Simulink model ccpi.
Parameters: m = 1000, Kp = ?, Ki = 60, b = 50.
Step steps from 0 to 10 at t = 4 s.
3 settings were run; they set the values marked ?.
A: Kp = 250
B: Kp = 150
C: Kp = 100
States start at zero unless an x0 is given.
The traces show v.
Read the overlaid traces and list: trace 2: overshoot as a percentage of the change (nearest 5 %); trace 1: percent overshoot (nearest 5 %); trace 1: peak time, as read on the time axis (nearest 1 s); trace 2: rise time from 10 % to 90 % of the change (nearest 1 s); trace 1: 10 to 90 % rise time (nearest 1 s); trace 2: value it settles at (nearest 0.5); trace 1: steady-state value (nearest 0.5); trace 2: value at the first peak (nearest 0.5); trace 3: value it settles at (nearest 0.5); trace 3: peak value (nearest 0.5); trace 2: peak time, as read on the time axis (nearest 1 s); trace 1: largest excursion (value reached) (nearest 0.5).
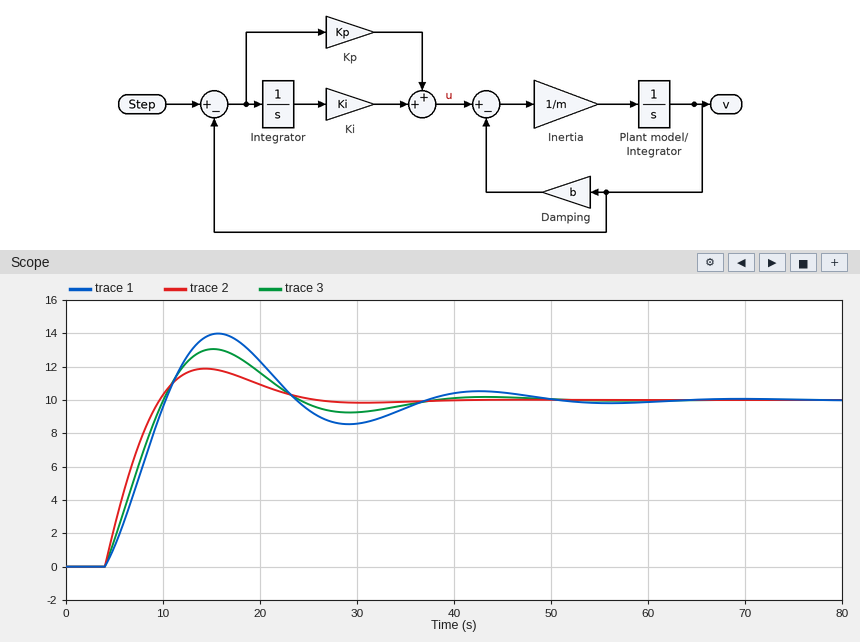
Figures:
20 %
40 %
16 s
4 s
5 s
10.0
10.0
12.0
10.0
13.0
14 s
14.0
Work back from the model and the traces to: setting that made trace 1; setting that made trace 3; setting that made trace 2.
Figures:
C
B
A
